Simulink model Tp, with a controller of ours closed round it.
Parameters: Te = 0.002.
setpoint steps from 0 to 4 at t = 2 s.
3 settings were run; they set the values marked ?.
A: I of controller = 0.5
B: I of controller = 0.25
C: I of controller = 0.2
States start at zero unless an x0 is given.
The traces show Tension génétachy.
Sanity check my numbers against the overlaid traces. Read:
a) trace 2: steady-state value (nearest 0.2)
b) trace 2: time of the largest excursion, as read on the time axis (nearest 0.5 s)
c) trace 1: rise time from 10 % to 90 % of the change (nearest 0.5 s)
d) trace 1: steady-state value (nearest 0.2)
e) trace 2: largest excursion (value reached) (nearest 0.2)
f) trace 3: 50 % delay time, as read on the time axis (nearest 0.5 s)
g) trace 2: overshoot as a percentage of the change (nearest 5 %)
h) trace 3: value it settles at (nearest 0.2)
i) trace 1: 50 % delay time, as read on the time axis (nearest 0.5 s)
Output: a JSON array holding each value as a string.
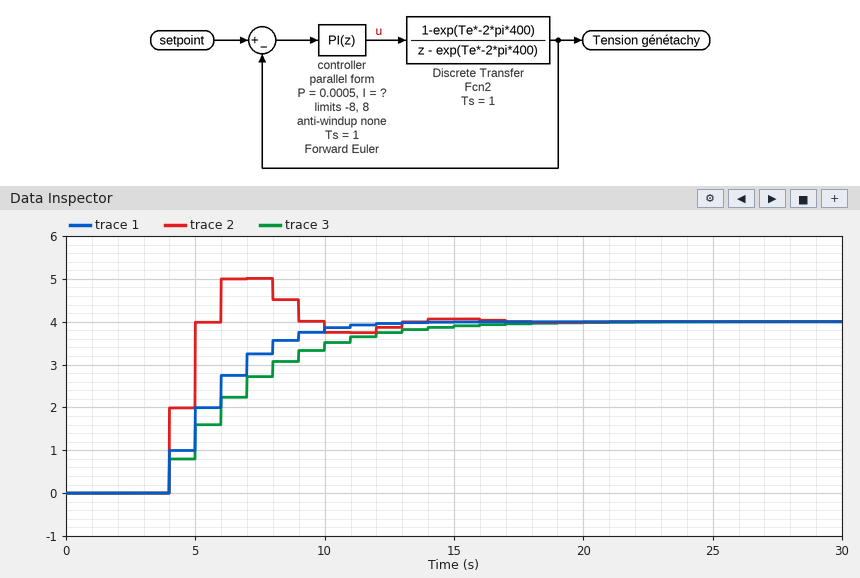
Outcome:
["4.0", "7.0 s", "5.0 s", "4.0", "5.0", "6.0 s", "25 %", "4.0", "6.0 s"]
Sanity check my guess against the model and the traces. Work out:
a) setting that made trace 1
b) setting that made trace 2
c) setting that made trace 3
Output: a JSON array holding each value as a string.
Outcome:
["B", "A", "C"]
